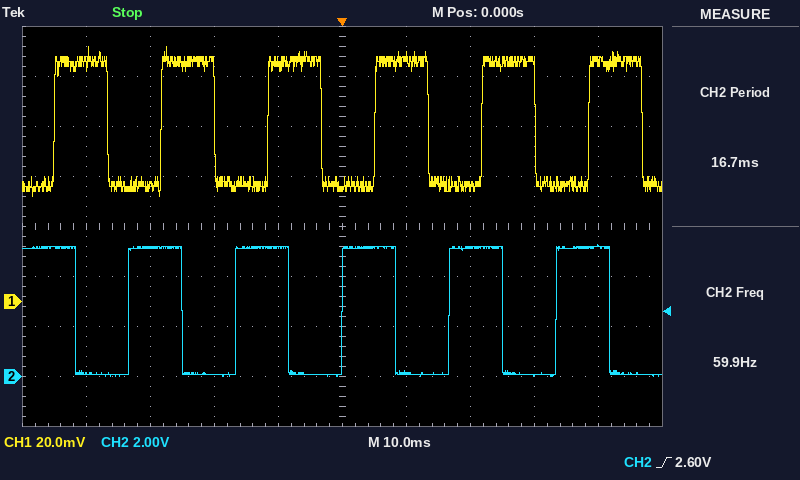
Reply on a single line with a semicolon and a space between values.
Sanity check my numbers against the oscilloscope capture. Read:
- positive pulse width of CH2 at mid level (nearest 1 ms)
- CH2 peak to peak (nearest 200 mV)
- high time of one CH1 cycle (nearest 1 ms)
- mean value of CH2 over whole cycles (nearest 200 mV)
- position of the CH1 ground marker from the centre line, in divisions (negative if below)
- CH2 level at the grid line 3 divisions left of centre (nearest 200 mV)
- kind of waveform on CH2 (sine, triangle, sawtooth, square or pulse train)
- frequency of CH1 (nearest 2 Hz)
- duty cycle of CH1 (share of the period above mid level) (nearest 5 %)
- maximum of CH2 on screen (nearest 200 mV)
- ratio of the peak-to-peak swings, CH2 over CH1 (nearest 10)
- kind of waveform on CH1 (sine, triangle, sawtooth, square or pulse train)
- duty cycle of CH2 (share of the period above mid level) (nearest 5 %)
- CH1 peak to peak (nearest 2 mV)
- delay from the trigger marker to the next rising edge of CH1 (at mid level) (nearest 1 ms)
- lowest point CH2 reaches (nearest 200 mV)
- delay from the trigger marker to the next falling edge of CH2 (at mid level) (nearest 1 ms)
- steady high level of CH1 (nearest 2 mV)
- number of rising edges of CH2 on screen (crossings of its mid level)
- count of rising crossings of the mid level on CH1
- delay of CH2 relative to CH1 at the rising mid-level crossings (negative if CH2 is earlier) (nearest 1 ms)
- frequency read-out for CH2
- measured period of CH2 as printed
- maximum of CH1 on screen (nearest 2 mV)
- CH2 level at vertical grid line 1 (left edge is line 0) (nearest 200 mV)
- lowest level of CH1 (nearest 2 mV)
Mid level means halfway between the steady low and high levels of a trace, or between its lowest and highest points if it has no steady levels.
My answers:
8 ms; 5.2 V; 8 ms; 2.6 V; -1.5 div; 5.2 V; square; 60 Hz; 50 %; 5.2 V; 90; square; 50 %; 60 mV; 5 ms; 0.0 V; 8 ms; 96 mV; 5; 6; -5 ms; 59.9 Hz; 16.7 ms; 102 mV; 200 mV; 42 mV
